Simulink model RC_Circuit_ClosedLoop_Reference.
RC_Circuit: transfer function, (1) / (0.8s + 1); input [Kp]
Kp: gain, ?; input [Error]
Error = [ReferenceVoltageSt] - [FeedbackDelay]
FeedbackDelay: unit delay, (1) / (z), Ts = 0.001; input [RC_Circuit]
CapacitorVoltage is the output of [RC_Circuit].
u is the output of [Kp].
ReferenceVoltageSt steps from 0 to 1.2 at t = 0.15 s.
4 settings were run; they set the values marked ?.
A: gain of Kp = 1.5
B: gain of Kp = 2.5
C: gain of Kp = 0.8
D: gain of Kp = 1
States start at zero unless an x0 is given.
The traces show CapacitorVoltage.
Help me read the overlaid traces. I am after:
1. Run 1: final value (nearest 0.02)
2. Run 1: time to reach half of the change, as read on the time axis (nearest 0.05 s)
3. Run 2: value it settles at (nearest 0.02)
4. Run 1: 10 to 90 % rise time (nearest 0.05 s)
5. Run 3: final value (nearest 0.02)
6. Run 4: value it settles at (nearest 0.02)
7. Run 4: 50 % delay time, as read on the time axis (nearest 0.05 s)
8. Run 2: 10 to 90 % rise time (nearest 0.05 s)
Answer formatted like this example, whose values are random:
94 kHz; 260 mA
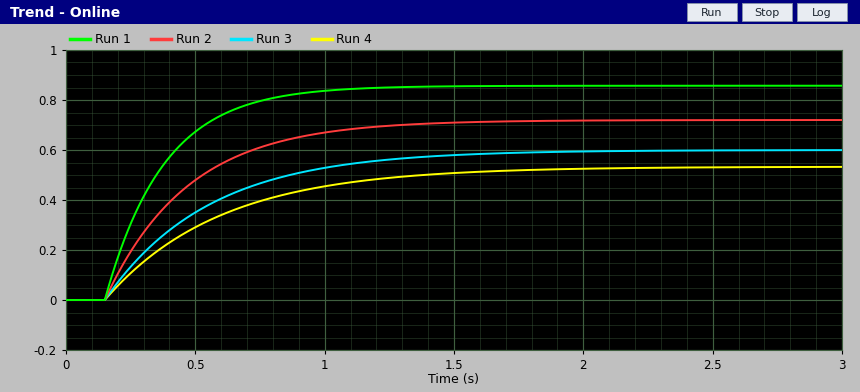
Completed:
0.86; 0.30 s; 0.72; 0.50 s; 0.60; 0.54; 0.45 s; 0.70 s
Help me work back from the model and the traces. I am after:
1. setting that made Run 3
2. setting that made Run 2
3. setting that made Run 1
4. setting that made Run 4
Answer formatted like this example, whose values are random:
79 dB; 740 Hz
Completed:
D; A; B; C
